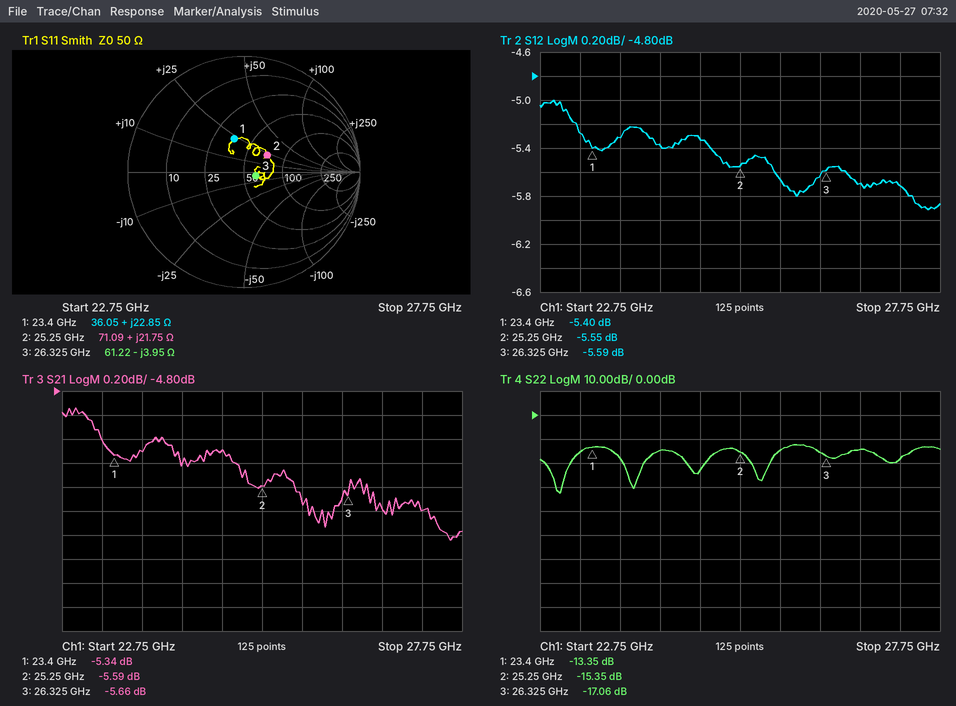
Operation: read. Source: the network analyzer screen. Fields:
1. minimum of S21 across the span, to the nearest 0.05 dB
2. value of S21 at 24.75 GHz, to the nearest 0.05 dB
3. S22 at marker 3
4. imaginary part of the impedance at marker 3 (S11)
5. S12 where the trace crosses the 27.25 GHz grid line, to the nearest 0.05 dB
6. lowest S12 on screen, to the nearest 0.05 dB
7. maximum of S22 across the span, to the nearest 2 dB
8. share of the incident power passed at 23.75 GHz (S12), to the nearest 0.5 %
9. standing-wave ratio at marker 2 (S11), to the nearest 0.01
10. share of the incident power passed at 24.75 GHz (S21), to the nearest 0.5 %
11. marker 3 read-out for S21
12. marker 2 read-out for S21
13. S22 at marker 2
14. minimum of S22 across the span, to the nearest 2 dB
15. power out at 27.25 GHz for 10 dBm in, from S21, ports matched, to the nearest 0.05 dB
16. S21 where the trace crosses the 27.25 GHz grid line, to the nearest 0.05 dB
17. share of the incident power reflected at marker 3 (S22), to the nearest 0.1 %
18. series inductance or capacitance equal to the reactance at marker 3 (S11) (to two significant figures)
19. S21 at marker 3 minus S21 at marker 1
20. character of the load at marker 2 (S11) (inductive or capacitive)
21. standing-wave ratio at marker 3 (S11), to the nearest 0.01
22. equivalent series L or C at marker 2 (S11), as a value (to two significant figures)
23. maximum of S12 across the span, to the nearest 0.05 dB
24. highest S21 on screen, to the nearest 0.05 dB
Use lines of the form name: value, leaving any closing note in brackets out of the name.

minimum of S21 across the span, to the nearest 0.05 dB: -6.05 dB
value of S21 at 24.75 GHz, to the nearest 0.05 dB: -5.30 dB
S22 at marker 3: -17.06 dB
imaginary part of the impedance at marker 3: -3.95 Ω
S12 where the trace crosses the 27.25 GHz grid line, to the nearest 0.05 dB: -5.70 dB
lowest S12 on screen, to the nearest 0.05 dB: -5.90 dB
maximum of S22 across the span, to the nearest 2 dB: -12 dB
share of the incident power passed at 23.75 GHz (S12), to the nearest 0.5 %: 29.5 %
standing-wave ratio at marker 2 (S11), to the nearest 0.01: 1.65
share of the incident power passed at 24.75 GHz (S21), to the nearest 0.5 %: 29.5 %
marker 3 read-out for S21: -5.66 dB
marker 2 read-out for S21: -5.59 dB
S22 at marker 2: -15.35 dB
minimum of S22 across the span, to the nearest 2 dB: -32 dB
power out at 27.25 GHz for 10 dBm in, from S21, ports matched, to the nearest 0.05 dB: 4.20 dBm
S21 where the trace crosses the 27.25 GHz grid line, to the nearest 0.05 dB: -5.80 dB
share of the incident power reflected at marker 3 (S22), to the nearest 0.1 %: 2.0 %
series inductance or capacitance equal to the reactance at marker 3 (S11): 1.5 pF
S21 at marker 3 minus S21 at marker 1: -0.32 dB
character of the load at marker 2 (S11): inductive
standing-wave ratio at marker 3 (S11), to the nearest 0.01: 1.24
equivalent series L or C at marker 2 (S11), as a value: 140 pH
maximum of S12 across the span, to the nearest 0.05 dB: -5.00 dB
highest S21 on screen, to the nearest 0.05 dB: -4.95 dB
